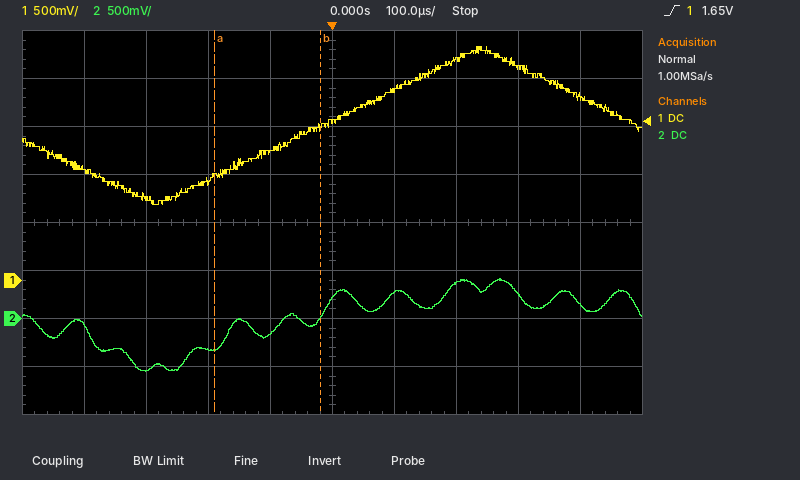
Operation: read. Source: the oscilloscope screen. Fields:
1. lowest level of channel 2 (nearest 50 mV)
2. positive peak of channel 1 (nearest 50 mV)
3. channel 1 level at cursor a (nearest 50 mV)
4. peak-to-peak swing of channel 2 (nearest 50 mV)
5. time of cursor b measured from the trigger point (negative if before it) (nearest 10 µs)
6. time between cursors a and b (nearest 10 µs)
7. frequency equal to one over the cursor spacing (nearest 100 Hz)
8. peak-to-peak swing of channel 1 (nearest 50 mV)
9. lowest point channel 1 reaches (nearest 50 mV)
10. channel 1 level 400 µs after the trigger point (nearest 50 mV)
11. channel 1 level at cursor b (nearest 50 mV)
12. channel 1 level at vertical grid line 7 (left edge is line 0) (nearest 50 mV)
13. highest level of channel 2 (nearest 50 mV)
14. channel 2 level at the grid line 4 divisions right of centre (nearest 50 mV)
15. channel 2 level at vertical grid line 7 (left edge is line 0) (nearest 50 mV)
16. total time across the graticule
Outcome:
-550 mV
2.45 V
1.10 V
950 mV
-20 µs
170 µs
5.9 kHz
1.65 V
800 mV
1.90 V
1.60 V
2.30 V
400 mV
150 mV
350 mV
1 ms
